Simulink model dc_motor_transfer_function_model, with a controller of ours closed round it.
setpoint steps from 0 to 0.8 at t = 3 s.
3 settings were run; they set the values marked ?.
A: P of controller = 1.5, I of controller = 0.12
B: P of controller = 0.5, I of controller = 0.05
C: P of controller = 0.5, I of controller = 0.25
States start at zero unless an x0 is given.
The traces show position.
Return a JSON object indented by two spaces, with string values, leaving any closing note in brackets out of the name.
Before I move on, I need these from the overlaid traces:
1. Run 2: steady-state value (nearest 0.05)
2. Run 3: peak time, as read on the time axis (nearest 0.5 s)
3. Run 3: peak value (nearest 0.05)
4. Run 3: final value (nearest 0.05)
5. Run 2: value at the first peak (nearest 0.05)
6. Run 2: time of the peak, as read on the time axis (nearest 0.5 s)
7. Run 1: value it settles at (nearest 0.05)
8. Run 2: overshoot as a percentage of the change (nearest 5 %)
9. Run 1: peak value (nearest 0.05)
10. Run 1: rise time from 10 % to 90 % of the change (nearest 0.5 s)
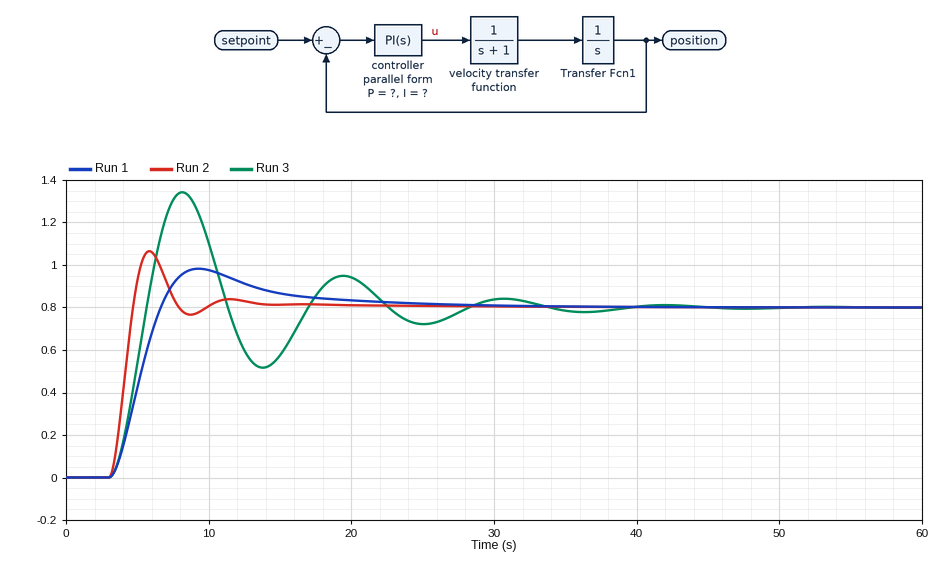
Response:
{
  "Run 2: steady-state value": "0.80",
  "Run 3: peak time, as read on the time axis": "8.0 s",
  "Run 3: peak value": "1.35",
  "Run 3: final value": "0.80",
  "Run 2: value at the first peak": "1.05",
  "Run 2: time of the peak, as read on the time axis": "6.0 s",
  "Run 1: value it settles at": "0.80",
  "Run 2: overshoot as a percentage of the change": "35 %",
  "Run 1: peak value": "1.00",
  "Run 1: rise time from 10 % to 90 % of the change": "2.5 s"
}
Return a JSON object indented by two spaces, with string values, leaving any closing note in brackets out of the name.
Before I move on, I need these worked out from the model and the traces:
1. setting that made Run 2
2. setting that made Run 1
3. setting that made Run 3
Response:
{
  "setting that made Run 2": "A",
  "setting that made Run 1": "B",
  "setting that made Run 3": "C"
}
